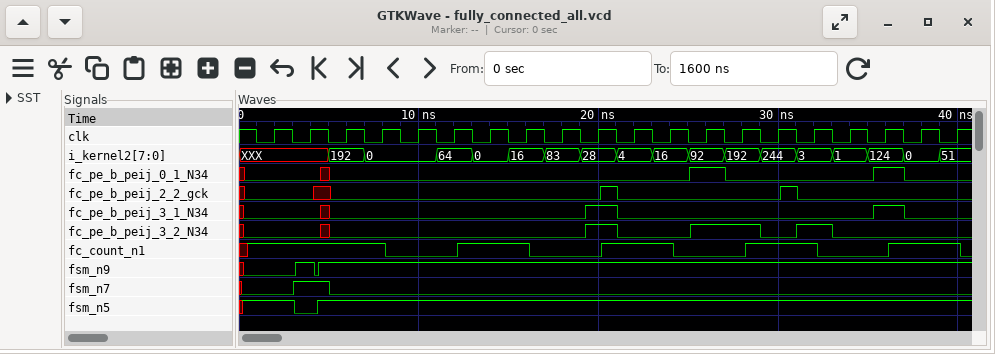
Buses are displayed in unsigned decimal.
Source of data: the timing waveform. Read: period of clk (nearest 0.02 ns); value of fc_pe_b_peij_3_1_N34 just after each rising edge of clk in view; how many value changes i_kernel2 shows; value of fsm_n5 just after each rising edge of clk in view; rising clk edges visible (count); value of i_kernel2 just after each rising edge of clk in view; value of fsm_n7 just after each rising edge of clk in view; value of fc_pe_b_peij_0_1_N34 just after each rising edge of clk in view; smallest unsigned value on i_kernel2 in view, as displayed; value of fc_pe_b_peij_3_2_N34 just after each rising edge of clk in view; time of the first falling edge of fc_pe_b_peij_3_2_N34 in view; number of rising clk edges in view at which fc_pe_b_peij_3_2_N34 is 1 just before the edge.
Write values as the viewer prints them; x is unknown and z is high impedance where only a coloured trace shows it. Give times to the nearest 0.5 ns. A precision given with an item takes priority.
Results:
2 ns
0 0 0 0 0 0 0 0 0 1 0 0 0 0 0 0 0 1 0 0
17
1 0 1 1 1 1 1 1 1 1 1 1 1 1 1 1 1 1 1 1
20
XXX, XXX, 192, 0, 0, 64, 0, 16, 83, 28, 4, 16, 92, 192, 244, 3, 1, 124, 0, 51
0 1 0 0 0 0 0 0 0 0 0 0 0 0 0 0 0 0 0 0
0 0 0 0 0 0 0 0 0 0 0 0 1 0 0 0 0 1 0 0
0
0 0 0 0 0 0 0 0 0 1 0 0 1 1 0 1 0 0 0 0
21 ns
4
